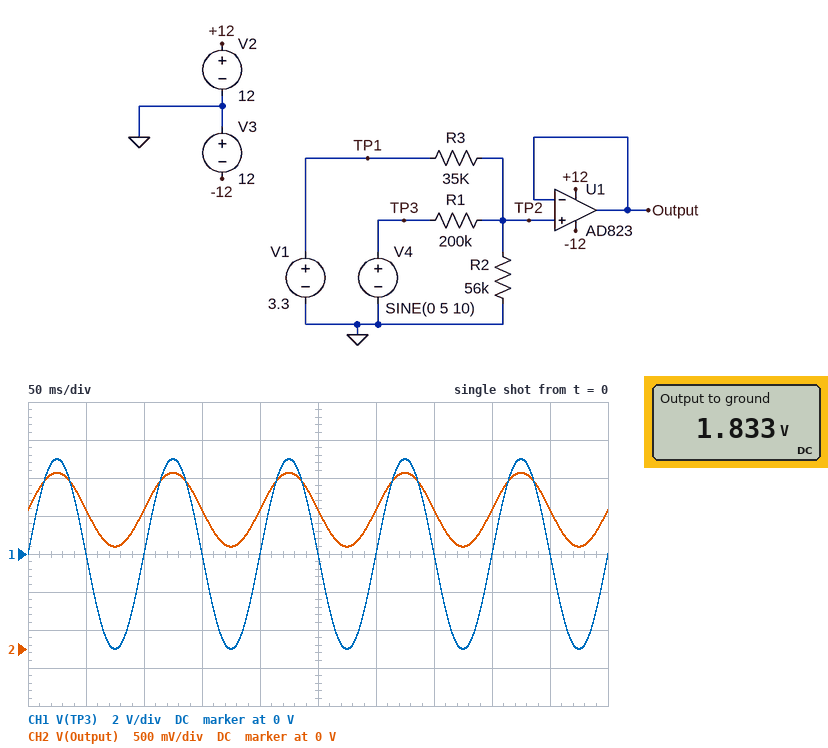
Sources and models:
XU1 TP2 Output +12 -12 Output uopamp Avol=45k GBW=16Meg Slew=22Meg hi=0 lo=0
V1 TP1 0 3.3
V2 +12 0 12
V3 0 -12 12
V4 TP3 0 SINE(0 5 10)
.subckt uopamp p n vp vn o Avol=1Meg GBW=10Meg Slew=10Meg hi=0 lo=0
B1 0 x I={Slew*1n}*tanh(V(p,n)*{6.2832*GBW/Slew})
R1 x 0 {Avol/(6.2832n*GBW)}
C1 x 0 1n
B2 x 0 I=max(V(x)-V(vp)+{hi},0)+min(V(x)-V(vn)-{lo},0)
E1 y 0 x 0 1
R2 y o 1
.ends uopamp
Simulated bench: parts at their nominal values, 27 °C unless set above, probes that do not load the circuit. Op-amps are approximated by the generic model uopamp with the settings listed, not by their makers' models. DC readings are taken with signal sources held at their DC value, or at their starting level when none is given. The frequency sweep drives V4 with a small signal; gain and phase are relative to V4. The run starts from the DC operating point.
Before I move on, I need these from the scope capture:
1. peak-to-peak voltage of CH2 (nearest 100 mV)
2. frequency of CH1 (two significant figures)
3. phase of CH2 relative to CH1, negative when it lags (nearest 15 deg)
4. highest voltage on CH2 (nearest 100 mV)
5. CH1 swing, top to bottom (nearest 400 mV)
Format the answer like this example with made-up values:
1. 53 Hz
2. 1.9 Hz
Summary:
1. 1.0 V
2. 10 Hz
3. 0 deg
4. 2.3 V
5. 10.0 V
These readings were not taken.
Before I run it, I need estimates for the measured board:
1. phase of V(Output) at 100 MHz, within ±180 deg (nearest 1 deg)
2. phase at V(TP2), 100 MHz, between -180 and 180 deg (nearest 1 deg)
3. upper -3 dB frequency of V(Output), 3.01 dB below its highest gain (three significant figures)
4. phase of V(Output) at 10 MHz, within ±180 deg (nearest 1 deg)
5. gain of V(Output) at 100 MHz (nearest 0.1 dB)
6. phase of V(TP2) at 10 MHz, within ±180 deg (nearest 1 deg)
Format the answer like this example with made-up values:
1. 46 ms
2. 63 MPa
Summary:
1. -81 deg
2. 0 deg
3. 16.0 MHz
4. -32 deg
5. -36.3 dB
6. 0 deg
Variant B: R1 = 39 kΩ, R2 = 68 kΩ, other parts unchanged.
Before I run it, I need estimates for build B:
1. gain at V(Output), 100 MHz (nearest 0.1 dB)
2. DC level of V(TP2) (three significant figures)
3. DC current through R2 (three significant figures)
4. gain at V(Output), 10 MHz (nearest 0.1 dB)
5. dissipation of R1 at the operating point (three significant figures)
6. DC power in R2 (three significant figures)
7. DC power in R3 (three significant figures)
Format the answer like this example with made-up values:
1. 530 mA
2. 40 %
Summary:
1. -24.6 dB
2. 1.37 V
3. 20.1 µA
4. -10.0 dB
5. 48.0 µW
6. 27.5 µW
7. 107 µW
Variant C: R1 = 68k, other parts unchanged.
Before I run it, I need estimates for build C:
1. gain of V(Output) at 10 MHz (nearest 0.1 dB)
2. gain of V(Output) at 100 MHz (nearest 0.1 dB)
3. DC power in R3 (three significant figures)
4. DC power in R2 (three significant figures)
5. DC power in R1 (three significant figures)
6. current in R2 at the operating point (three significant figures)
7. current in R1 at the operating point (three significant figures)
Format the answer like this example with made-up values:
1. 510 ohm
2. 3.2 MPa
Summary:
1. -13.8 dB
2. -28.4 dB
3. 88.3 µW
4. 42.5 µW
5. 35.0 µW
6. 27.5 µA
7. 22.7 µA
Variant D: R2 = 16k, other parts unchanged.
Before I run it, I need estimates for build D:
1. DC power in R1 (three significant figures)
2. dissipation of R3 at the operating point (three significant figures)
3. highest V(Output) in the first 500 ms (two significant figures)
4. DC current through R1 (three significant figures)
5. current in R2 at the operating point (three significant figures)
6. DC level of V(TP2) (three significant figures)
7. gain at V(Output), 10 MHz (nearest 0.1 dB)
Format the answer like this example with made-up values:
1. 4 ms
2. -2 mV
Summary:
1. 4.82 µW
2. 154 µW
3. 1.2 V
4. 4.91 µA
5. 61.3 µA
6. 981 mV
7. -27.1 dB
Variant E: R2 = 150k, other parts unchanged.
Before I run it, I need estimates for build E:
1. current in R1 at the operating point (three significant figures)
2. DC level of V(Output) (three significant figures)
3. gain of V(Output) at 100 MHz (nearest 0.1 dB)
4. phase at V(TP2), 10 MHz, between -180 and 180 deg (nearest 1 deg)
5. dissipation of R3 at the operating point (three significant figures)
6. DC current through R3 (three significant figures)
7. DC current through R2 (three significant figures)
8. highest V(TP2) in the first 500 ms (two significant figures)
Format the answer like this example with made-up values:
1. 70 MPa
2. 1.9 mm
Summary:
1. 11.7 µA
2. 2.34 V
3. -34.1 dB
4. 0 deg
5. 26.2 µW
6. 27.3 µA
7. 15.6 µA
8. 3.0 V
